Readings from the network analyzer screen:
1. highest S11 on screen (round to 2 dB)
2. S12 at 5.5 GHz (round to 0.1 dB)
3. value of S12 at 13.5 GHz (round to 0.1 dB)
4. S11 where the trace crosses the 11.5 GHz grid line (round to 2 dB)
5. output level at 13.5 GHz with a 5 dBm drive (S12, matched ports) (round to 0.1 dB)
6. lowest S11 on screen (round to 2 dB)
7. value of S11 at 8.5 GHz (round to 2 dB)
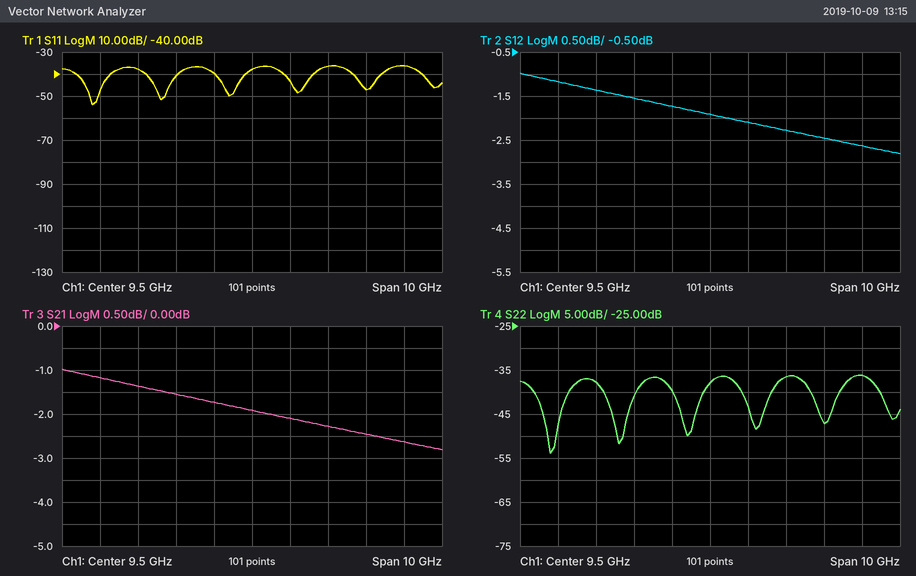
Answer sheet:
-36 dB
-1.2 dB
-2.6 dB
-36 dB
2.4 dBm
-54 dB
-40 dB
